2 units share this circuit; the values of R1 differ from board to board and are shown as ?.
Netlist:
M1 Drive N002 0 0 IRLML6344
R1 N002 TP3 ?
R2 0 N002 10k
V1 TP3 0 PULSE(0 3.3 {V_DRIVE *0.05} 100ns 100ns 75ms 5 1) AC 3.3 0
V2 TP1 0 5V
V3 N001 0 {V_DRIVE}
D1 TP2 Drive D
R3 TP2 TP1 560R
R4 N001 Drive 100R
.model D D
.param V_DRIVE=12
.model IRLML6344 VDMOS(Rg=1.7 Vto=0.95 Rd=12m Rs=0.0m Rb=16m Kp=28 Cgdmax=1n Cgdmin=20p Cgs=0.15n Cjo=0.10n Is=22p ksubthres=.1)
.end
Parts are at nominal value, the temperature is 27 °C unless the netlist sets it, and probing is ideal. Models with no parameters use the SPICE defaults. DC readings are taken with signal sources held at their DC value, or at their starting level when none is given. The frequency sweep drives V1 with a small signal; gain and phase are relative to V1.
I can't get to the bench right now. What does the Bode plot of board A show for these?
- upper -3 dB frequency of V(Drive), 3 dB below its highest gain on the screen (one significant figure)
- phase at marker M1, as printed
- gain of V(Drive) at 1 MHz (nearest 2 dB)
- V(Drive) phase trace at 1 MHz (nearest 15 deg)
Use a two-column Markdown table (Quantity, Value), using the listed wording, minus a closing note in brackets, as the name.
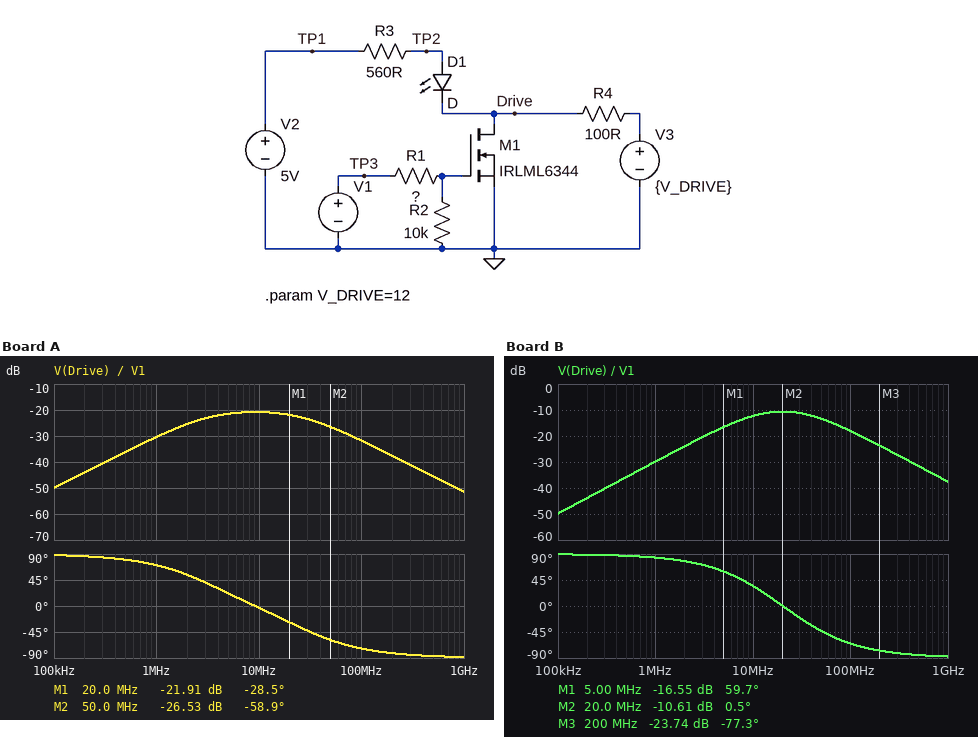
| Quantity | Value |
|---|---|
| upper -3 dB frequency of V(Drive), 3 dB below its highest gain on the screen | 30 MHz |
| phase at marker M1, as printed | -28.5 deg |
| gain of V(Drive) at 1 MHz | -30 dB |
| V(Drive) phase trace at 1 MHz | 75 deg |
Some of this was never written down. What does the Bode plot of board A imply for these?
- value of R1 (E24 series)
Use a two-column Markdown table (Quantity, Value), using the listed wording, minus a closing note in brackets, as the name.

| Quantity | Value |
|---|---|
| value of R1 | 240 Ω |
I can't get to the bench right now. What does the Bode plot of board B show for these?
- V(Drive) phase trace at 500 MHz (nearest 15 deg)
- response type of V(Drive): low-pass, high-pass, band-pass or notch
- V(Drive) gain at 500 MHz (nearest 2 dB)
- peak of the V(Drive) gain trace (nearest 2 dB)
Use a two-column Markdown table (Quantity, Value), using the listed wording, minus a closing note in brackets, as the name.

| Quantity | Value |
|---|---|
| V(Drive) phase trace at 500 MHz | -90 deg |
| response type of V(Drive): low-pass, high-pass, band-pass or notch | band-pass |
| V(Drive) gain at 500 MHz | -32 dB |
| peak of the V(Drive) gain trace | -10 dB |
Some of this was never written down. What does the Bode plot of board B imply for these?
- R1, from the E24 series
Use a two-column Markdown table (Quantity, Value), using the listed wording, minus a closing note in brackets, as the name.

| Quantity | Value |
|---|---|
| R1, from the E24 series | 47 Ω |
